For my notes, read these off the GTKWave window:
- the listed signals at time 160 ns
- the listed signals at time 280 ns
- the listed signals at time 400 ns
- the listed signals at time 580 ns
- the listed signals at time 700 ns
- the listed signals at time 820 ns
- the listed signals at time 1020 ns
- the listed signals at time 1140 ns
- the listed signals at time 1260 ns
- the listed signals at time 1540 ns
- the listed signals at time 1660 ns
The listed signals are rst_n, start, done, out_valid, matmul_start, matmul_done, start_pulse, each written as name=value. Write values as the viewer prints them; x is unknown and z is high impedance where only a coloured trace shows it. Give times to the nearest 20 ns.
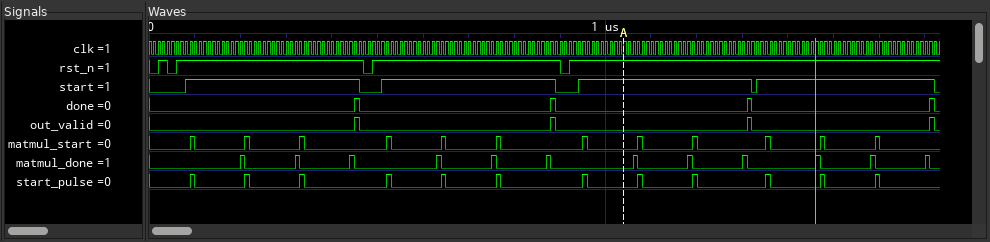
rst_n=1, start=1, done=0, out_valid=0, matmul_start=0, matmul_done=0, start_pulse=0
rst_n=1, start=1, done=0, out_valid=0, matmul_start=0, matmul_done=0, start_pulse=0
rst_n=1, start=1, done=0, out_valid=0, matmul_start=0, matmul_done=0, start_pulse=0
rst_n=1, start=1, done=0, out_valid=0, matmul_start=0, matmul_done=0, start_pulse=0
rst_n=1, start=1, done=0, out_valid=0, matmul_start=0, matmul_done=0, start_pulse=0
rst_n=1, start=1, done=0, out_valid=0, matmul_start=0, matmul_done=0, start_pulse=0
rst_n=1, start=1, done=0, out_valid=0, matmul_start=0, matmul_done=0, start_pulse=0
rst_n=1, start=1, done=0, out_valid=0, matmul_start=0, matmul_done=0, start_pulse=0
rst_n=1, start=1, done=0, out_valid=0, matmul_start=0, matmul_done=0, start_pulse=0
rst_n=1, start=1, done=0, out_valid=0, matmul_start=0, matmul_done=0, start_pulse=0
rst_n=1, start=1, done=0, out_valid=0, matmul_start=0, matmul_done=0, start_pulse=0
